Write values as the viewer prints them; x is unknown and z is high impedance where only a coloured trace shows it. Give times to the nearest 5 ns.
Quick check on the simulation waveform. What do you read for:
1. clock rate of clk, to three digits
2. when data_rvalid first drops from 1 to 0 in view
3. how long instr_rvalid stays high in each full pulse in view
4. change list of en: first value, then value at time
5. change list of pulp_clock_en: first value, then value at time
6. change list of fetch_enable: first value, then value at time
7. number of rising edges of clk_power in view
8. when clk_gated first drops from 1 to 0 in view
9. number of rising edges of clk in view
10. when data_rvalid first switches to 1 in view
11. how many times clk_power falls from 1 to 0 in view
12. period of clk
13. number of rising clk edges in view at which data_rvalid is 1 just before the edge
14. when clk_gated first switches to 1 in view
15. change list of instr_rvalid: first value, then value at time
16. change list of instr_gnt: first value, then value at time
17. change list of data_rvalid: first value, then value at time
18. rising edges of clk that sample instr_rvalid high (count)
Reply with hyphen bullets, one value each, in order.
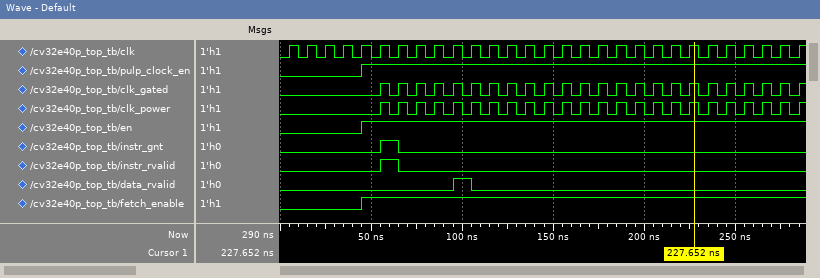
- 100 MHz
- 105 ns
- 10 ns
- 0, 1 at 45 ns
- 0, 1 at 45 ns
- 0, 1 at 45 ns
- 24
- 60 ns
- 29
- 95 ns
- 23
- 10 ns
- 1
- 55 ns
- 0, 1 at 55 ns, 0 at 65 ns
- 0, 1 at 55 ns, 0 at 65 ns
- 0, 1 at 95 ns, 0 at 105 ns
- 1
